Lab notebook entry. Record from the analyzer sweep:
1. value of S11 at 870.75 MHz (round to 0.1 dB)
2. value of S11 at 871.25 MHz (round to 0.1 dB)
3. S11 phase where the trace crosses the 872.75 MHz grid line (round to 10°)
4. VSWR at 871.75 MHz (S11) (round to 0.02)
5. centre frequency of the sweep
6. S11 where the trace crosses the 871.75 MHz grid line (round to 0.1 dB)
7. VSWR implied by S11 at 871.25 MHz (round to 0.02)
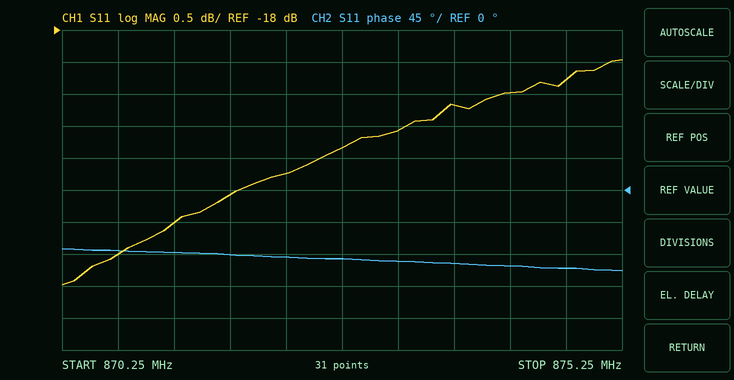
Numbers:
-21.5 dB
-21.0 dB
-100°
1.20
872.75 MHz
-20.6 dB
1.20
